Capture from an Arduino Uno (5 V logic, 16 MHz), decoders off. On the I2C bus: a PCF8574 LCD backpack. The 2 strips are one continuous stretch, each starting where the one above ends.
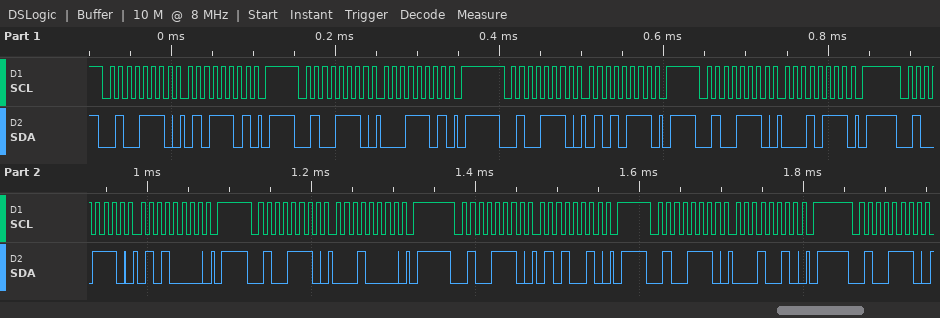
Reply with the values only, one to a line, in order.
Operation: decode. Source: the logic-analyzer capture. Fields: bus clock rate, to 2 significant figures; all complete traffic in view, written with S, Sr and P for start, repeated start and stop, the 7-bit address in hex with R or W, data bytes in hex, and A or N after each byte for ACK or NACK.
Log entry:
100 kHz
S 27W A 5D A P S 27W A 1D A P S 27W A 57 A P S 27W A 17 A P S 27W A 50 A P S 27W A 10 A P S 27W A 52 A P S 27W A 12 A P S 27W A
